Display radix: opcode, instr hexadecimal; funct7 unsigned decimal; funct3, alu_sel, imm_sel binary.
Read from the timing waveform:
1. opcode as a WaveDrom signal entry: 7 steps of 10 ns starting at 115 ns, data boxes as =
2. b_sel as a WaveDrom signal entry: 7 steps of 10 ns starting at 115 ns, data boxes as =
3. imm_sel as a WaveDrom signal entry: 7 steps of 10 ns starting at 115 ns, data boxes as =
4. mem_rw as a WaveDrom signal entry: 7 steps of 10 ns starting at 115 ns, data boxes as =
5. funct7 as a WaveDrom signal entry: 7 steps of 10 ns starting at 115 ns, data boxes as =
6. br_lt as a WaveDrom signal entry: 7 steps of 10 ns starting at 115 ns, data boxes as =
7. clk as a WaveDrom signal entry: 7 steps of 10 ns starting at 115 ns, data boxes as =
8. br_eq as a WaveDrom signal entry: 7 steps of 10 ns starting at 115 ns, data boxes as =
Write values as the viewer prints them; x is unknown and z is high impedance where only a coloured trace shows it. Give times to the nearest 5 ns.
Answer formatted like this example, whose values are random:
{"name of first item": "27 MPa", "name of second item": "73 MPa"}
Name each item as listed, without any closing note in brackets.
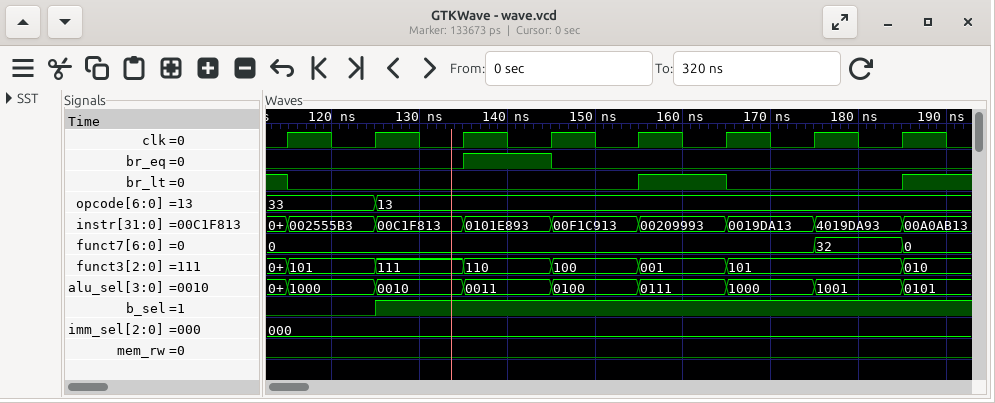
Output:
{"opcode as a WaveDrom signal entry: 7 steps of 10 ns starting at 115 ns, data boxes as =": "{name: 'opcode', wave: '==.....', data: '33 13'}", "b_sel as a WaveDrom signal entry: 7 steps of 10 ns starting at 115 ns, data boxes as =": "{name: 'b_sel', wave: '01.....'}", "imm_sel as a WaveDrom signal entry: 7 steps of 10 ns starting at 115 ns, data boxes as =": "{name: 'imm_sel', wave: '=......', data: '000'}", "mem_rw as a WaveDrom signal entry: 7 steps of 10 ns starting at 115 ns, data boxes as =": "{name: 'mem_rw', wave: '0......'}", "funct7 as a WaveDrom signal entry: 7 steps of 10 ns starting at 115 ns, data boxes as =": "{name: 'funct7', wave: '=.....=', data: '0 32'}", "br_lt as a WaveDrom signal entry: 7 steps of 10 ns starting at 115 ns, data boxes as =": "{name: 'br_lt', wave: '0...10.'}", "clk as a WaveDrom signal entry: 7 steps of 10 ns starting at 115 ns, data boxes as =": "{name: 'clk', wave: 'p......'}", "br_eq as a WaveDrom signal entry: 7 steps of 10 ns starting at 115 ns, data boxes as =": "{name: 'br_eq', wave: '0.10...'}"}
